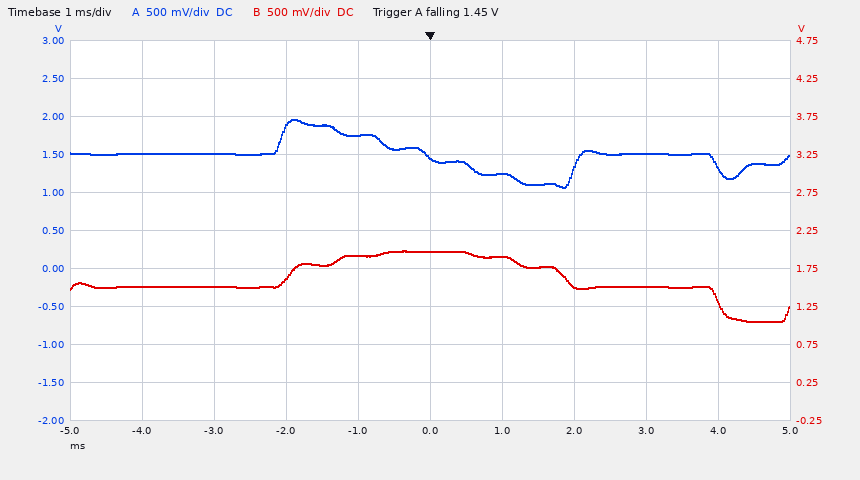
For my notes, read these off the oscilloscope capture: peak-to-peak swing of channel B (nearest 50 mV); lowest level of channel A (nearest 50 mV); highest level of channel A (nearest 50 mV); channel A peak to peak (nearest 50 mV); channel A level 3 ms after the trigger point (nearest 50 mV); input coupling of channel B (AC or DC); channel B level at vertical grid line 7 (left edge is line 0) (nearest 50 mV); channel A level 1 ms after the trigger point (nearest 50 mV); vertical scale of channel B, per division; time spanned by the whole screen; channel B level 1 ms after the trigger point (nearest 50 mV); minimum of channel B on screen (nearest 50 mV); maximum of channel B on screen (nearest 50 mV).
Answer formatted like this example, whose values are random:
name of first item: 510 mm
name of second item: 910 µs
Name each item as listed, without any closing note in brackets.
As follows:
peak-to-peak swing of channel B: 950 mV
lowest level of channel A: 1.05 V
highest level of channel A: 1.95 V
channel A peak to peak: 900 mV
channel A level 3 ms after the trigger point: 1.50 V
input coupling of channel B: DC
channel B level at vertical grid line 7 (left edge is line 0): 1.50 V
channel A level 1 ms after the trigger point: 1.25 V
vertical scale of channel B, per division: 500 mV
time spanned by the whole screen: 10 ms
channel B level 1 ms after the trigger point: 1.90 V
minimum of channel B on screen: 1.05 V
maximum of channel B on screen: 2.00 V
